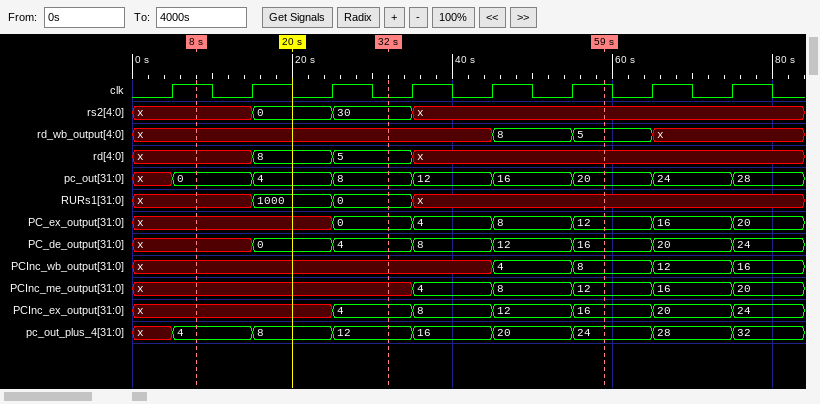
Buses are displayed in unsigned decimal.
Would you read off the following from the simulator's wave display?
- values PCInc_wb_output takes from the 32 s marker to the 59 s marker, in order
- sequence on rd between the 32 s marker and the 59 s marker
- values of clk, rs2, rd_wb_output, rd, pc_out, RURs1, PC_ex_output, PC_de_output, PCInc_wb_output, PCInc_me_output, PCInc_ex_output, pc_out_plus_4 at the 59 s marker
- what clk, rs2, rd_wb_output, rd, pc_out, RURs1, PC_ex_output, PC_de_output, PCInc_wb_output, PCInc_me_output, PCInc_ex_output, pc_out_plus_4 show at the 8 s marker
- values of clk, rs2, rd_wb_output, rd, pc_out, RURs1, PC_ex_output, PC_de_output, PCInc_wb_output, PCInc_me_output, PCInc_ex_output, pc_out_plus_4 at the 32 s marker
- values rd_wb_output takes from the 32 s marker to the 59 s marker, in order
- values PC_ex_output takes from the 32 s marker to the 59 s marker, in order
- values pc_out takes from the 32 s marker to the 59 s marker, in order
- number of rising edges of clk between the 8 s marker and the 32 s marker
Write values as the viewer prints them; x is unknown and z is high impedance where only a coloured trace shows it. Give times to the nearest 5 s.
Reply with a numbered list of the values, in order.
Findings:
1. x, 4, 8
2. 5, x
3. clk=1, rs2=x, rd_wb_output=5, rd=x, pc_out=20, RURs1=x, PC_ex_output=12, PC_de_output=16, PCInc_wb_output=8, PCInc_me_output=12, PCInc_ex_output=16, pc_out_plus_4=24
4. clk=1, rs2=x, rd_wb_output=x, rd=x, pc_out=0, RURs1=x, PC_ex_output=x, PC_de_output=x, PCInc_wb_output=x, PCInc_me_output=x, PCInc_ex_output=x, pc_out_plus_4=4
5. clk=0, rs2=30, rd_wb_output=x, rd=5, pc_out=8, RURs1=0, PC_ex_output=0, PC_de_output=4, PCInc_wb_output=x, PCInc_me_output=x, PCInc_ex_output=4, pc_out_plus_4=12
6. x, 8, 5
7. 0, 4, 8, 12
8. 8, 12, 16, 20
9. 2
